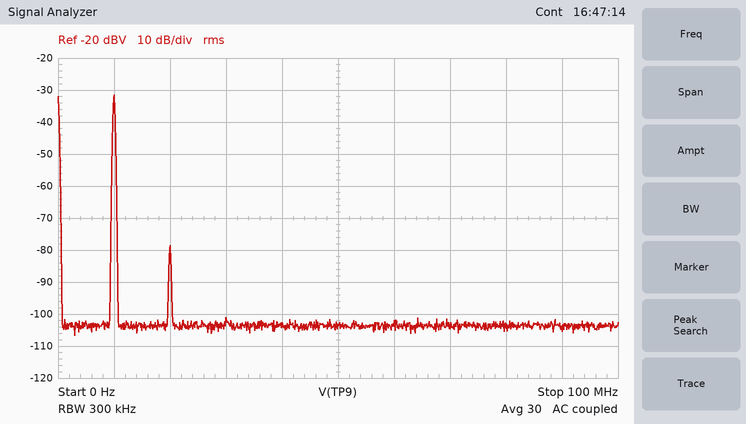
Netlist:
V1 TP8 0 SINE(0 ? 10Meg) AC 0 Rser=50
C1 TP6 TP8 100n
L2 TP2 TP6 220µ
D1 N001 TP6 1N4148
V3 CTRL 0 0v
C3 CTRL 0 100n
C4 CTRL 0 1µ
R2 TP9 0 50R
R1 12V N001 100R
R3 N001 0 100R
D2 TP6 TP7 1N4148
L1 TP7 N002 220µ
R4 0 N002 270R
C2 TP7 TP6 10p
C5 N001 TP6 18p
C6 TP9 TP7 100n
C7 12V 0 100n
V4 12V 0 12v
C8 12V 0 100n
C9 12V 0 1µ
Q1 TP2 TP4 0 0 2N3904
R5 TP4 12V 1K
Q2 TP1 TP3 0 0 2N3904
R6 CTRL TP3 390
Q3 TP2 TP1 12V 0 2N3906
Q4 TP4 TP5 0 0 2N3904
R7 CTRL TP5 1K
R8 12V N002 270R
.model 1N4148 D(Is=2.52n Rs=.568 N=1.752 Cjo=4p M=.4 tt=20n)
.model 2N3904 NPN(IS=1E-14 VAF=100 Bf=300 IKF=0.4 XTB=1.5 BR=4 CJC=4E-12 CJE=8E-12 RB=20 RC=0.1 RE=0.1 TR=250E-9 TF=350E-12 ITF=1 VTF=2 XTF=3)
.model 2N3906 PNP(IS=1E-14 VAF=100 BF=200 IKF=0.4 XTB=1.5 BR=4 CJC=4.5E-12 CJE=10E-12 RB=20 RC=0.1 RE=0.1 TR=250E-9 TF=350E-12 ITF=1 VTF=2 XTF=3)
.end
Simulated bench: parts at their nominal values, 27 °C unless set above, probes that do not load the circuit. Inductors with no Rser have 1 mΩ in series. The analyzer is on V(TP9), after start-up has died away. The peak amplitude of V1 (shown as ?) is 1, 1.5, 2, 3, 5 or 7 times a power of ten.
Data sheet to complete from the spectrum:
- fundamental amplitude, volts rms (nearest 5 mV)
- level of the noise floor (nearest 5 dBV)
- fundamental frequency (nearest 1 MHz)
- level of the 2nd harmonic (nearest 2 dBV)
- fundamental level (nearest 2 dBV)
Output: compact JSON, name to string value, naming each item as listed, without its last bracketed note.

{"fundamental amplitude, volts rms": "25 mV", "level of the noise floor": "-105 dBV", "fundamental frequency": "10 MHz", "level of the 2nd harmonic": "-78 dBV", "fundamental level": "-32 dBV"}
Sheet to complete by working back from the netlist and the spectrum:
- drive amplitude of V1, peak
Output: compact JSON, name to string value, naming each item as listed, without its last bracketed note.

{"drive amplitude of V1, peak": "2 V"}
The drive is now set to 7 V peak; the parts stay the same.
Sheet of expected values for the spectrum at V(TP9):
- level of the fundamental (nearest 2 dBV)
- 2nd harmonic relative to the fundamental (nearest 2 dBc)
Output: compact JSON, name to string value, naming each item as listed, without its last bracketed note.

{"level of the fundamental": "-20 dBV", "2nd harmonic relative to the fundamental": "-36 dBc"}
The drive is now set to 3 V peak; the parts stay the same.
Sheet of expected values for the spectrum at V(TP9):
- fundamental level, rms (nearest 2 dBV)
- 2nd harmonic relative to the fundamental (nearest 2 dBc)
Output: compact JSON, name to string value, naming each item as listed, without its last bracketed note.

{"fundamental level, rms": "-28 dBV", "2nd harmonic relative to the fundamental": "-44 dBc"}
